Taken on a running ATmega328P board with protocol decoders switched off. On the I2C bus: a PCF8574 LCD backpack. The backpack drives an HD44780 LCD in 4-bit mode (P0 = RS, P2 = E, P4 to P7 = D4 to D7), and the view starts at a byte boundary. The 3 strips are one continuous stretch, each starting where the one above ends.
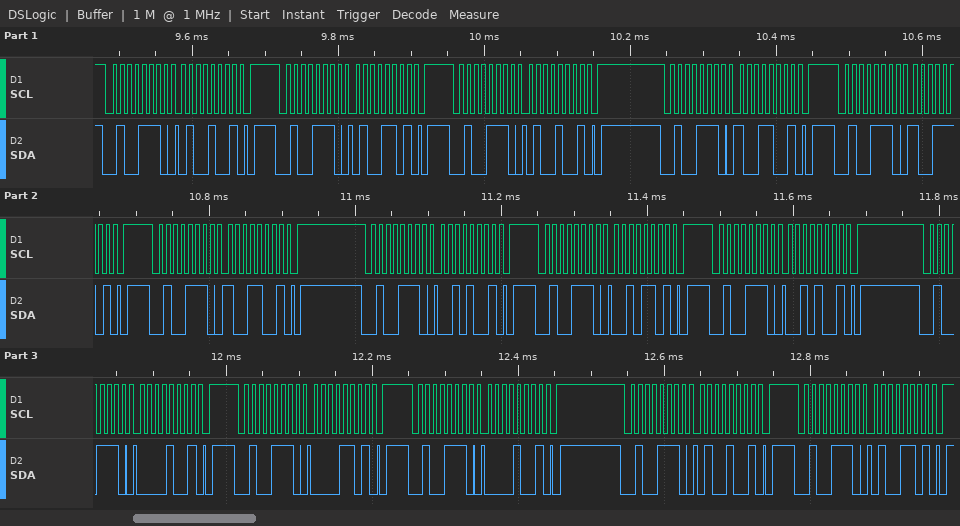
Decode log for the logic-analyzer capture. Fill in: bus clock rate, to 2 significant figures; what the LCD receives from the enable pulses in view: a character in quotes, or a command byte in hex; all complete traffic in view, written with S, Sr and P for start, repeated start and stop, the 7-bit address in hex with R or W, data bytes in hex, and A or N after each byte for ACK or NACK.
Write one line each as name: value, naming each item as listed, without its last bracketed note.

bus clock rate, to 2 significant figures: 100 kHz
what the LCD receives from the enable pulses in view: a character in quotes, or a command byte in hex: 'I' ' '
all complete traffic in view, written with S, Sr and P for start, repeated start and stop, the 7-bit address in hex with R or W, data bytes in hex, and A or N after each byte for ACK or NACK: S 27W A 49 A P S 27W A 4D A P S 27W A 49 A P S 27W A 99 A P S 27W A 9D A P S 27W A 99 A P S 27W A 29 A P S 27W A 2D A P S 27W A 29 A P S 27W A 09 A P S 27W A 0D A P S 27W A 09 A P S 27W A 49 A P S 27W A 4D A P
